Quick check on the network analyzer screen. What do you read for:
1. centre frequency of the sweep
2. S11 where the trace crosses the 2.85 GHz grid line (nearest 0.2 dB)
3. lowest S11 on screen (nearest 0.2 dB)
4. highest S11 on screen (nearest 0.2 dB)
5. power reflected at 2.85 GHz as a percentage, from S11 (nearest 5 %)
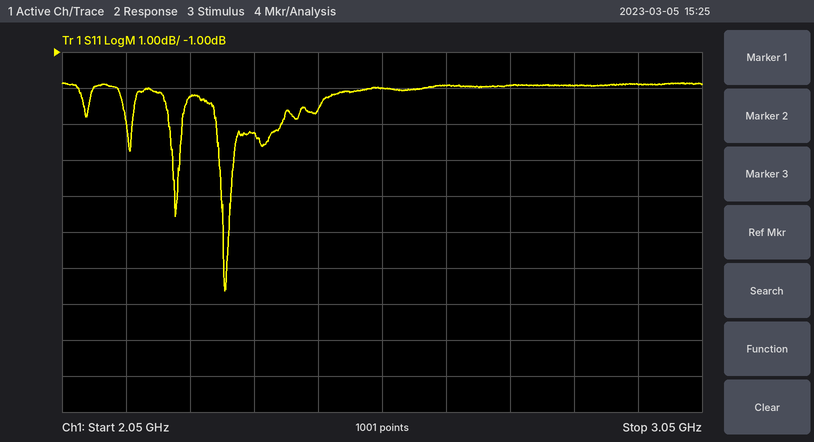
2.55 GHz
-2.0 dB
-7.6 dB
-1.8 dB
65 %
